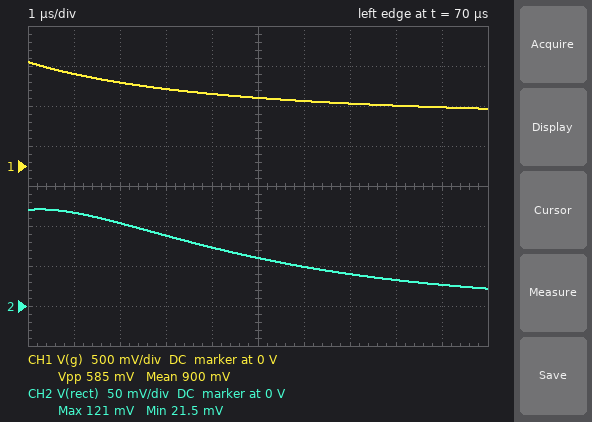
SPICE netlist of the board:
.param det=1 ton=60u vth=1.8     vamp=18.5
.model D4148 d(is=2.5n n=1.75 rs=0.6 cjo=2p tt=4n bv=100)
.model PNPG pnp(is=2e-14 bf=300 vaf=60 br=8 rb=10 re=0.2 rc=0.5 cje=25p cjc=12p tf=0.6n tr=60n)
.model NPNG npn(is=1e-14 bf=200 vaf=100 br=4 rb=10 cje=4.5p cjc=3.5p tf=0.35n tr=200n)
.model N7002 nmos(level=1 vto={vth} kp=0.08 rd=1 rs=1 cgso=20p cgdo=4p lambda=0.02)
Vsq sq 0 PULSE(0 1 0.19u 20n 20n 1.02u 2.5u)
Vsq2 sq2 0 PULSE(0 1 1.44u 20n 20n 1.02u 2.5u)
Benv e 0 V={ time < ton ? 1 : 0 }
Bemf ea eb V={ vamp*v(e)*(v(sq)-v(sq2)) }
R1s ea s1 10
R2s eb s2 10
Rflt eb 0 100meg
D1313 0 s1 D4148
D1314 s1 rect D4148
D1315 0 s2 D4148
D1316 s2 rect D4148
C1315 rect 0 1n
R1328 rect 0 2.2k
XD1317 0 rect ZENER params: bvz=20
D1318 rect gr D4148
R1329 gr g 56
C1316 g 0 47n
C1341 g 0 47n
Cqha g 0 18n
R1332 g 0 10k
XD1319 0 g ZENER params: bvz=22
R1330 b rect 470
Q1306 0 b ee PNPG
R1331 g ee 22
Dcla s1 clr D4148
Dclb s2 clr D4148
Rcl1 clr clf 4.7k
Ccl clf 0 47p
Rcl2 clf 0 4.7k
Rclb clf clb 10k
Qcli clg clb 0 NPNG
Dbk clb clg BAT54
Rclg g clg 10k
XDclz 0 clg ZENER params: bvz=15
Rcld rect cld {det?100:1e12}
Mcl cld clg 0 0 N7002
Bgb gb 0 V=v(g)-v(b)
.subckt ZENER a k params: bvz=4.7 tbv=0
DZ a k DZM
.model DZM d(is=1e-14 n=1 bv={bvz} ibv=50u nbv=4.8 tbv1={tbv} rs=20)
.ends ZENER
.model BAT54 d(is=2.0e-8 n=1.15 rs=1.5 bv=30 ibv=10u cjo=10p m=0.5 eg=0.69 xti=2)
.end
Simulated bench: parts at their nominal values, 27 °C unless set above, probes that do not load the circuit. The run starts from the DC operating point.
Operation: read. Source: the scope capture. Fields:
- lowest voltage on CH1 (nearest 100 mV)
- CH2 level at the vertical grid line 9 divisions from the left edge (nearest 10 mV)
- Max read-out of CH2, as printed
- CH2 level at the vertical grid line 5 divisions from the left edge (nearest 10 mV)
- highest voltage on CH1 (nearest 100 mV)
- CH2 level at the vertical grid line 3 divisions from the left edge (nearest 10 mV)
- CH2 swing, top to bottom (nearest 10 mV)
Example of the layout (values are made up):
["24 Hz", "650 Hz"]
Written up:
["700 mV", "30 mV", "121 mV", "60 mV", "1.3 V", "90 mV", "100 mV"]
